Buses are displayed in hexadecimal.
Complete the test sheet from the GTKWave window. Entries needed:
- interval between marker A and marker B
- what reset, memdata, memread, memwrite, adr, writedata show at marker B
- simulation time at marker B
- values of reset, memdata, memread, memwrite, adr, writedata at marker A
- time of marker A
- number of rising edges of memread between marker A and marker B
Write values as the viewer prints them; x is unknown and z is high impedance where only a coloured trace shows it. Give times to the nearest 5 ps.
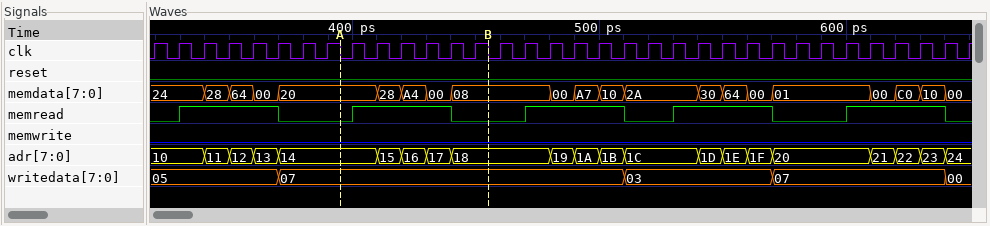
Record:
60 ps
reset=0, memdata=08, memread=0, memwrite=0, adr=18, writedata=07
455 ps
reset=0, memdata=20, memread=0, memwrite=0, adr=14, writedata=07
395 ps
1
